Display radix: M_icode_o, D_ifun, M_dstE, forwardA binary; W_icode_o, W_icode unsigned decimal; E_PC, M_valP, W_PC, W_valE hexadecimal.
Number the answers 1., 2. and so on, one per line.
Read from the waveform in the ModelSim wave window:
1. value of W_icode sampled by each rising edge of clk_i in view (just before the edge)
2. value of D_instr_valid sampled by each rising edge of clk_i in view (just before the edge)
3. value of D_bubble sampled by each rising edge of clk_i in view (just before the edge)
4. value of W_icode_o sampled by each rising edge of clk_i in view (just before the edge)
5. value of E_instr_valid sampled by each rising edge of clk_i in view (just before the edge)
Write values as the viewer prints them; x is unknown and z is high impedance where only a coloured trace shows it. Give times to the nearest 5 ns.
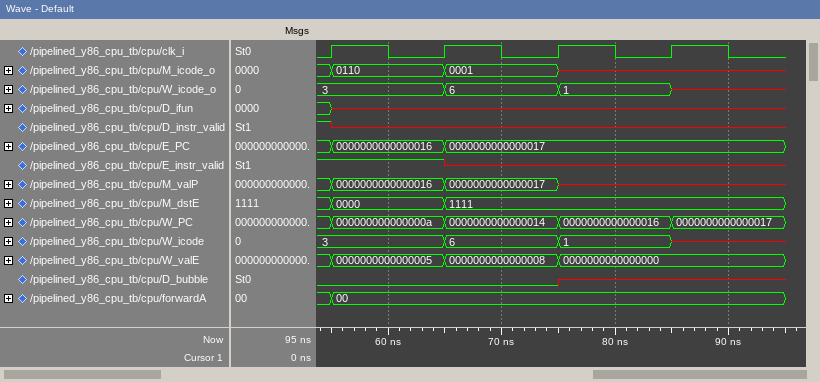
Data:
1. 3, 3, 6, 1
2. 1 x x x
3. 0 0 0 x
4. 3, 3, 6, 1
5. 1 1 x x
